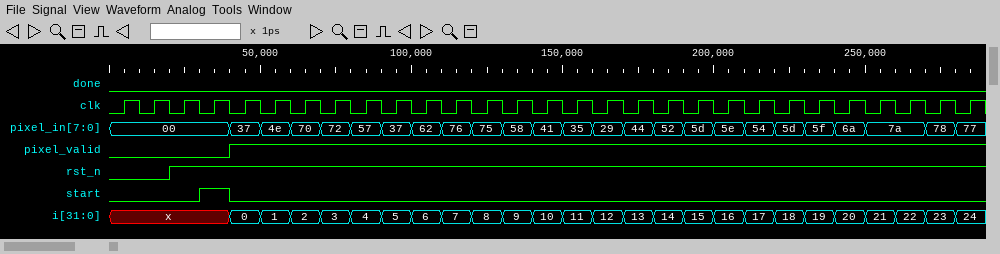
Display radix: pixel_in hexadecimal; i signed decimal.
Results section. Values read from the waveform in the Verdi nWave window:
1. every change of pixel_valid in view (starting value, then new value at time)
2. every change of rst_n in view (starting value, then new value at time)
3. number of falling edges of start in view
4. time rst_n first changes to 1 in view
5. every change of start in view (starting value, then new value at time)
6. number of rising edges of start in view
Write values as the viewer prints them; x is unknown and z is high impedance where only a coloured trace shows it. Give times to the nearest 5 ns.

0, 1 at 40 ns
0, 1 at 20 ns
1
20 ns
0, 1 at 30 ns, 0 at 40 ns
1
